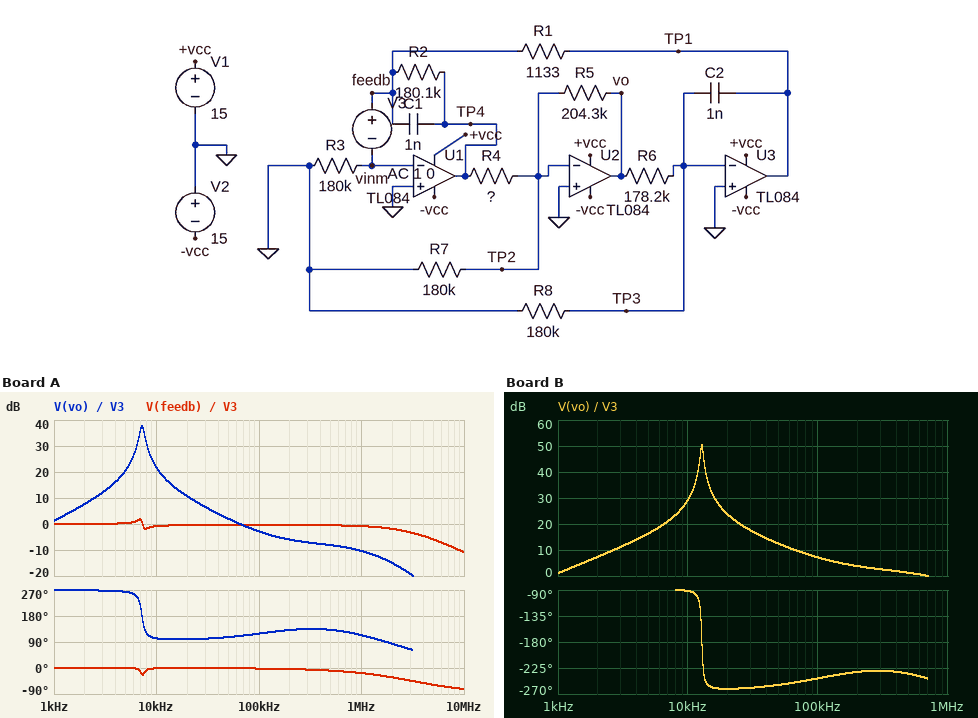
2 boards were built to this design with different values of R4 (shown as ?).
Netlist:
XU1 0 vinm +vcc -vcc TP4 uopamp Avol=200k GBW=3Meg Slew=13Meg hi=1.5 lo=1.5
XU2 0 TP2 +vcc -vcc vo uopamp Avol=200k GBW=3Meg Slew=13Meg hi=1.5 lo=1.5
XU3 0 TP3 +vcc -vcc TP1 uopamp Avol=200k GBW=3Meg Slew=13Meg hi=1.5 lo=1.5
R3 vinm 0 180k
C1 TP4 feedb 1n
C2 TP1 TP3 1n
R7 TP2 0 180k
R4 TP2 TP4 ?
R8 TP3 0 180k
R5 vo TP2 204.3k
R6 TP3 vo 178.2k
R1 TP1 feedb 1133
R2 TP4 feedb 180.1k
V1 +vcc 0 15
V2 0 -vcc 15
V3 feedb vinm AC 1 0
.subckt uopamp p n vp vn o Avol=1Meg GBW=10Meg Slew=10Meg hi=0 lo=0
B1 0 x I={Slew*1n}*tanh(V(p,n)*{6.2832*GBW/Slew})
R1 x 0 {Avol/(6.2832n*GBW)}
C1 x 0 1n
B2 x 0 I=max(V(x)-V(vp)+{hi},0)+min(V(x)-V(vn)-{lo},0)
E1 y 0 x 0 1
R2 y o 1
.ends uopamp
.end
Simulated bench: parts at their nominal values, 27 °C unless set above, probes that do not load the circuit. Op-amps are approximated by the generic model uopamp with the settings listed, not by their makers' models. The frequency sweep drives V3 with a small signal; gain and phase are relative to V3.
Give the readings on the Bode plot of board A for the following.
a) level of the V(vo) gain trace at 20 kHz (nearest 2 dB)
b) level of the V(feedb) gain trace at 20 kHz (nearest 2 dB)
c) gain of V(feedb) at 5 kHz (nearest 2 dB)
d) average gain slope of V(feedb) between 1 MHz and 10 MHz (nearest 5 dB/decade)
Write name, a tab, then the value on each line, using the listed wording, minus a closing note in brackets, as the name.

level of the V(vo) gain trace at 20 kHz	10 dB
level of the V(feedb) gain trace at 20 kHz	0 dB
gain of V(feedb) at 5 kHz	0 dB
average gain slope of V(feedb) between 1 MHz and 10 MHz	-10 dB/decade
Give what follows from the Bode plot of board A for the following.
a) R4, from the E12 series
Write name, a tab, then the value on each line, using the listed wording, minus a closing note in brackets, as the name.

R4, from the E12 series	470 kΩ
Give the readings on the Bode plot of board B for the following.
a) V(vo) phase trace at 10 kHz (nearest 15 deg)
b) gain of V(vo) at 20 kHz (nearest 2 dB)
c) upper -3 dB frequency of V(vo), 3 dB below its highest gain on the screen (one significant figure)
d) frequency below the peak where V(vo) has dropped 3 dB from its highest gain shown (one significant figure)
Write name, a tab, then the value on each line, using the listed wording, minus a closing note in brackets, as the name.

V(vo) phase trace at 10 kHz	-90 deg
gain of V(vo) at 20 kHz	24 dB
upper -3 dB frequency of V(vo), 3 dB below its highest gain on the screen	10 kHz
frequency below the peak where V(vo) has dropped 3 dB from its highest gain shown	10 kHz
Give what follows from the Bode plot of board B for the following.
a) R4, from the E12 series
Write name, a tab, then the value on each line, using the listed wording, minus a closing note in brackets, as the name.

R4, from the E12 series	150 kΩ
